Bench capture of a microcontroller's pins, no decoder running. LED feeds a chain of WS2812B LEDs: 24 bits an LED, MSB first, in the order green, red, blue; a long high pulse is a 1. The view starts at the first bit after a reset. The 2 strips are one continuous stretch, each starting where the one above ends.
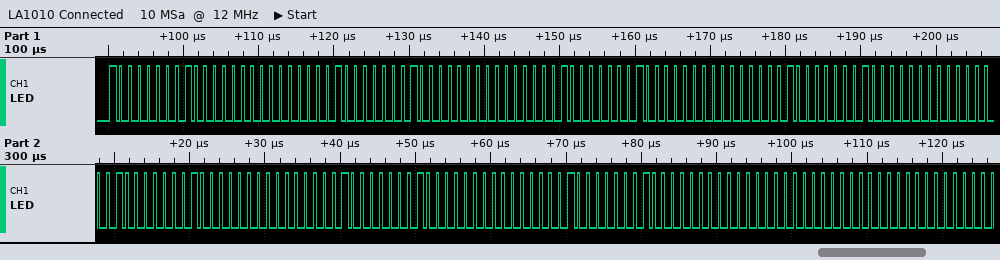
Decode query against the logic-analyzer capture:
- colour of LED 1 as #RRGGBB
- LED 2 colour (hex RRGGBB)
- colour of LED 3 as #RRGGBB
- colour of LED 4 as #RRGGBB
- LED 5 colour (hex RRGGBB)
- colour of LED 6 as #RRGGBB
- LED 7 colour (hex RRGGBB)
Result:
#808000
#808000
#808000
#808000
#808000
#808000
#808000
